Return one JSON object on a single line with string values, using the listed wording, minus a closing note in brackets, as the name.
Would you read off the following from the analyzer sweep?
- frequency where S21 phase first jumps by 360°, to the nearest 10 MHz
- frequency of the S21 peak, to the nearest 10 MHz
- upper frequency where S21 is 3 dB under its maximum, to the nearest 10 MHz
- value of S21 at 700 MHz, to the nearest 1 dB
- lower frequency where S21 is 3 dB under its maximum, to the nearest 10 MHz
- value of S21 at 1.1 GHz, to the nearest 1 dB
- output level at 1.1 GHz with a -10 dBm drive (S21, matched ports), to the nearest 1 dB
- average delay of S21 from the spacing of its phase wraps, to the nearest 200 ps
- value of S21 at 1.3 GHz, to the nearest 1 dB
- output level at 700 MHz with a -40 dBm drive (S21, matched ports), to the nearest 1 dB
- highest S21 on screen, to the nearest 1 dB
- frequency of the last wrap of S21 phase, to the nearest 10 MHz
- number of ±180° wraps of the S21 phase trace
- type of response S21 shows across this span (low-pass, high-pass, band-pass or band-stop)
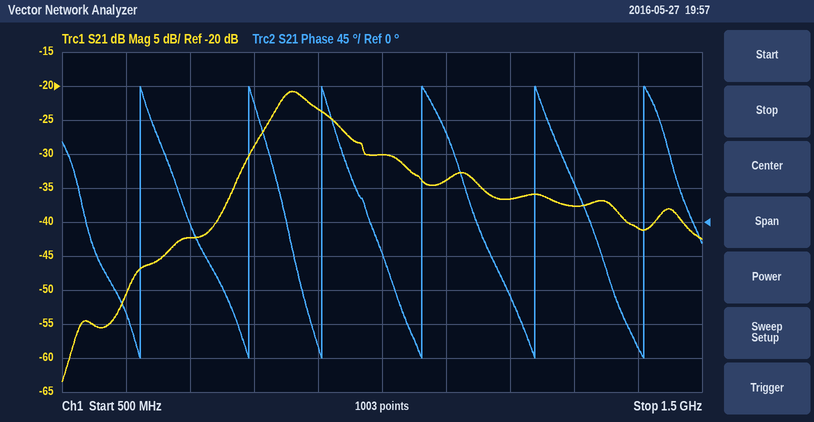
{"frequency where S21 phase first jumps by 360°, to the nearest 10 MHz": "620 MHz", "frequency of the S21 peak, to the nearest 10 MHz": "860 MHz", "upper frequency where S21 is 3 dB under its maximum, to the nearest 10 MHz": "910 MHz", "value of S21 at 700 MHz, to the nearest 1 dB": "-42 dB", "lower frequency where S21 is 3 dB under its maximum, to the nearest 10 MHz": "830 MHz", "value of S21 at 1.1 GHz, to the nearest 1 dB": "-34 dB", "output level at 1.1 GHz with a -10 dBm drive (S21, matched ports), to the nearest 1 dB": "-44 dBm", "average delay of S21 from the spacing of its phase wraps, to the nearest 200 ps": "6.4 ns", "value of S21 at 1.3 GHz, to the nearest 1 dB": "-38 dB", "output level at 700 MHz with a -40 dBm drive (S21, matched ports), to the nearest 1 dB": "-82 dBm", "highest S21 on screen, to the nearest 1 dB": "-21 dB", "frequency of the last wrap of S21 phase, to the nearest 10 MHz": "1.41 GHz", "number of ±180° wraps of the S21 phase trace": "6", "type of response S21 shows across this span": "band-pass"}
